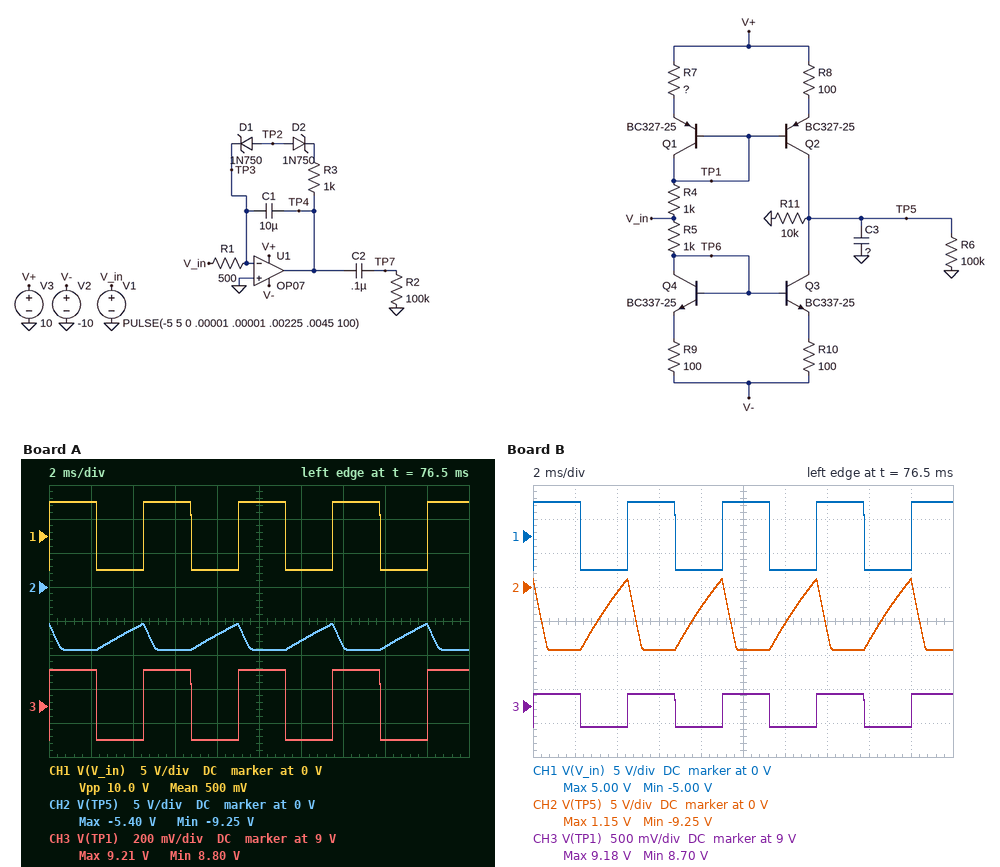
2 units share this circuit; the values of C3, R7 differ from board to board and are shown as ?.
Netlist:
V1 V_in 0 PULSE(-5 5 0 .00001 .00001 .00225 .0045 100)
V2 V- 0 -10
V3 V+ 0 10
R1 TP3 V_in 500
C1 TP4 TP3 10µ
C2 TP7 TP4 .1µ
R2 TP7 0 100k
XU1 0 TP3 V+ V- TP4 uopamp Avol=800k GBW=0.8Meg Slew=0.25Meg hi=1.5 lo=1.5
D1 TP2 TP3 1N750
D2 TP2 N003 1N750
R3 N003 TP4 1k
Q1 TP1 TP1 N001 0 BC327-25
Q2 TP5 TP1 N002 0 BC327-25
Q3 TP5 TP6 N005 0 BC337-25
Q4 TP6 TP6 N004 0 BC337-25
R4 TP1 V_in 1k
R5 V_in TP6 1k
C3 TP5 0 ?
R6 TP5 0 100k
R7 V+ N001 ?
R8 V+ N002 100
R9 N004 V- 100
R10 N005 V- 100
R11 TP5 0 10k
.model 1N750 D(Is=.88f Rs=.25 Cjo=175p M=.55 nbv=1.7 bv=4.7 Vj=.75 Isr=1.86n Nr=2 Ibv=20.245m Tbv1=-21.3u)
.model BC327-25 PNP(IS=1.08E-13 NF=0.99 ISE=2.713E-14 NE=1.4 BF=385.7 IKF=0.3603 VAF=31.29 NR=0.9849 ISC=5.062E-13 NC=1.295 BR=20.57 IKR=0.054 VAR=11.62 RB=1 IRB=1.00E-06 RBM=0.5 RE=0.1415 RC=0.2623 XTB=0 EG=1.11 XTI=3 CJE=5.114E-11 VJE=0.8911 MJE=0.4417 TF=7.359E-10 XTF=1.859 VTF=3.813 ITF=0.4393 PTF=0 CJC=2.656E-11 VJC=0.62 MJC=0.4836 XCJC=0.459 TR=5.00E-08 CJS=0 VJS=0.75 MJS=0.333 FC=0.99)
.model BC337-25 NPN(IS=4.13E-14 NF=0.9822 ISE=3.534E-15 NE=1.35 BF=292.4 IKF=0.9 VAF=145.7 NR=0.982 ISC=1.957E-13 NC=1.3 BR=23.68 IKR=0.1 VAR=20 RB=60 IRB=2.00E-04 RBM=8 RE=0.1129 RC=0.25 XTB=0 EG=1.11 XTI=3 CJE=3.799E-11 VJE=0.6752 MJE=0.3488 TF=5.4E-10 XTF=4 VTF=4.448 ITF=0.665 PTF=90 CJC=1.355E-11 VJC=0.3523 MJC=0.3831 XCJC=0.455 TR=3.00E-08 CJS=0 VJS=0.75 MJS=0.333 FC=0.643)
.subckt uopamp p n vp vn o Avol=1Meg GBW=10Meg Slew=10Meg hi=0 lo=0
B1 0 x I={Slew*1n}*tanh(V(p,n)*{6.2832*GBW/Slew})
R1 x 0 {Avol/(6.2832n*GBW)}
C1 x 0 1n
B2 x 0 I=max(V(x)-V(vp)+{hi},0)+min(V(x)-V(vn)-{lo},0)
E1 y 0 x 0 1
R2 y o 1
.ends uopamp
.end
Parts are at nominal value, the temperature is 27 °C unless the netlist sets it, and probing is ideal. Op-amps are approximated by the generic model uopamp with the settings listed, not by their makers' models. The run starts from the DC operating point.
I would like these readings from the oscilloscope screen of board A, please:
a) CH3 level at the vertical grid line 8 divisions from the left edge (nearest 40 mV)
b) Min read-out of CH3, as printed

8.80 V
8.80 V
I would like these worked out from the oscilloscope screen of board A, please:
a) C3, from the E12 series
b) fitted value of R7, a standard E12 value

1.5 µF
39 Ω
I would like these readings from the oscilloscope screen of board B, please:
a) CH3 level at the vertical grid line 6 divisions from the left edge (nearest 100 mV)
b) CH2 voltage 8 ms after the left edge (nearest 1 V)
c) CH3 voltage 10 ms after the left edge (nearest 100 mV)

8.7 V
-3 V
9.2 V
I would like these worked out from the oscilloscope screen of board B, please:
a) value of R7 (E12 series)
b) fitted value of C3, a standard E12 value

47 Ω
680 nF
